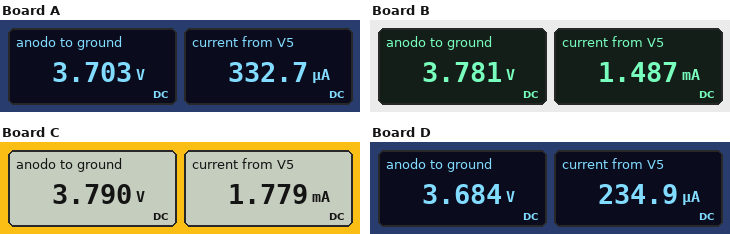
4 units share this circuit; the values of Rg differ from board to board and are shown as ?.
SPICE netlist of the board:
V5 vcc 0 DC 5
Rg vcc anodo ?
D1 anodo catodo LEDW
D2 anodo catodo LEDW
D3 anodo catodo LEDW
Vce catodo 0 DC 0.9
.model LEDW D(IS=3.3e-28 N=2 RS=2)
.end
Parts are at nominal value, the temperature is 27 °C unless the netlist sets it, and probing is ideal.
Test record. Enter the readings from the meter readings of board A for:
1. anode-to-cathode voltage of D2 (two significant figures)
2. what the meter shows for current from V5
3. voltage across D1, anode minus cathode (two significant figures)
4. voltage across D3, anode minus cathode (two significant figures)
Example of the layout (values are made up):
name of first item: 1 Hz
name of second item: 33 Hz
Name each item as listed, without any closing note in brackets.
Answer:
anode-to-cathode voltage of D2: 2.8 V
what the meter shows for current from V5: 332.7 µA
voltage across D1, anode minus cathode: 2.8 V
voltage across D3, anode minus cathode: 2.8 V
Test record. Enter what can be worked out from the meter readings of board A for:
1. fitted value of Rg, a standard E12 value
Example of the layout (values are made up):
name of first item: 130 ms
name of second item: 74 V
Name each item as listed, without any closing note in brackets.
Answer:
fitted value of Rg, a standard E12 value: 3.9 kΩ
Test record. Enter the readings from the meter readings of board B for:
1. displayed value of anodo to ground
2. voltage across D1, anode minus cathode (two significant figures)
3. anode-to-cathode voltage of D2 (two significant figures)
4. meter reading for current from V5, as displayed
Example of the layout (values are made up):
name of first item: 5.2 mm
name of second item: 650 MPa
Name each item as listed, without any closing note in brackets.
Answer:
displayed value of anodo to ground: 3.781 V
voltage across D1, anode minus cathode: 2.9 V
anode-to-cathode voltage of D2: 2.9 V
meter reading for current from V5, as displayed: 1.487 mA
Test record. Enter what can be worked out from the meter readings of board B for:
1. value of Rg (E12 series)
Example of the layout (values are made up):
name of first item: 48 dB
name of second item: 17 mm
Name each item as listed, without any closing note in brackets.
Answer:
value of Rg: 820 Ω
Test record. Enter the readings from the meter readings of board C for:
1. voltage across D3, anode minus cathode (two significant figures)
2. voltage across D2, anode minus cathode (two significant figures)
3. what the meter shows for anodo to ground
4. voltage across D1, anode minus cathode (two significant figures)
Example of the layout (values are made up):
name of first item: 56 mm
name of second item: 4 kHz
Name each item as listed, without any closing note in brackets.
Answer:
voltage across D3, anode minus cathode: 2.9 V
voltage across D2, anode minus cathode: 2.9 V
what the meter shows for anodo to ground: 3.790 V
voltage across D1, anode minus cathode: 2.9 V
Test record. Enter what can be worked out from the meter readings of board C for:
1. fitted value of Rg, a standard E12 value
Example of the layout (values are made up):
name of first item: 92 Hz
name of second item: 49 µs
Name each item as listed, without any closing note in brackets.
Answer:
fitted value of Rg, a standard E12 value: 680 Ω
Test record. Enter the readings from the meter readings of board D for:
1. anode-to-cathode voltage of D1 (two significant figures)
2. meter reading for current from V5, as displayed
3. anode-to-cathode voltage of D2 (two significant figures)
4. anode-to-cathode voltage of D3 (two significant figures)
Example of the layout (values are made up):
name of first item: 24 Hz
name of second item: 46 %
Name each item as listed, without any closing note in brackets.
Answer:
anode-to-cathode voltage of D1: 2.8 V
meter reading for current from V5, as displayed: 234.9 µA
anode-to-cathode voltage of D2: 2.8 V
anode-to-cathode voltage of D3: 2.8 V
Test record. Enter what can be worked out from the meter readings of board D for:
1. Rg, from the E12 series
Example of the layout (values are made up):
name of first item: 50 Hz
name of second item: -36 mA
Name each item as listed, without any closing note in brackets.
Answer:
Rg, from the E12 series: 5.6 kΩ
